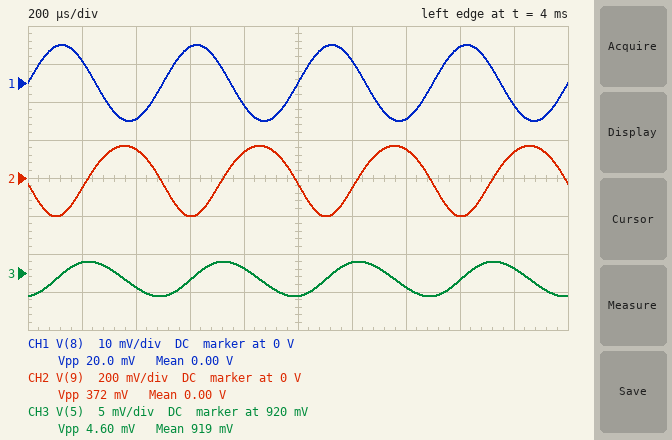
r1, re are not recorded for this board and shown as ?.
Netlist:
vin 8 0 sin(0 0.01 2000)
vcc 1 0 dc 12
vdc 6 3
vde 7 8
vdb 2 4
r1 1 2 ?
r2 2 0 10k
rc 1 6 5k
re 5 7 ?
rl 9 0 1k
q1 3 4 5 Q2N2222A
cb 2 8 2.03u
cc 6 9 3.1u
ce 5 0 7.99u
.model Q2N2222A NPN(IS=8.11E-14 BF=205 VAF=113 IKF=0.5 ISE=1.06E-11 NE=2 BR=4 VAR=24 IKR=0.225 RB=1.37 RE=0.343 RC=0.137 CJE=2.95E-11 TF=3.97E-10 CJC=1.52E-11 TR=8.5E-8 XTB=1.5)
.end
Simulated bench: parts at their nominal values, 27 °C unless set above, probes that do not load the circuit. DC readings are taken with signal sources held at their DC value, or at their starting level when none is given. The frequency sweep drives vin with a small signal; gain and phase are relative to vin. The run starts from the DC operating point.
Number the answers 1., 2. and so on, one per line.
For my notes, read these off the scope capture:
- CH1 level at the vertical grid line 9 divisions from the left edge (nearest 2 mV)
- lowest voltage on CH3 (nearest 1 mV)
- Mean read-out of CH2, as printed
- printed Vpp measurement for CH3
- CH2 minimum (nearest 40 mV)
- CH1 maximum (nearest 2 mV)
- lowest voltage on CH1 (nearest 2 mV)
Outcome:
1. -6 mV
2. 917 mV
3. 0.00 V
4. 4.60 mV
5. -200 mV
6. 10 mV
7. -10 mV
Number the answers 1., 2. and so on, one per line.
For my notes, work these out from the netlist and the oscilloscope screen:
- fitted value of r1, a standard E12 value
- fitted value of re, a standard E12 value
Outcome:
1. 68 kΩ
2. 1.5 kΩ
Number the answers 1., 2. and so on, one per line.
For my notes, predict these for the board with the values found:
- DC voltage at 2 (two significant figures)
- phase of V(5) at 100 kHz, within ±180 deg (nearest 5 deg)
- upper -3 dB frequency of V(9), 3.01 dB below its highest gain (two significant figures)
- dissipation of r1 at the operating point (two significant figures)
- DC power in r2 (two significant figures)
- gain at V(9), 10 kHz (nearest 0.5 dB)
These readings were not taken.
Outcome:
1. 1.5 V
2. -90 deg
3. 27 MHz
4. 1.6 mW
5. 230 µW
6. 25.5 dB
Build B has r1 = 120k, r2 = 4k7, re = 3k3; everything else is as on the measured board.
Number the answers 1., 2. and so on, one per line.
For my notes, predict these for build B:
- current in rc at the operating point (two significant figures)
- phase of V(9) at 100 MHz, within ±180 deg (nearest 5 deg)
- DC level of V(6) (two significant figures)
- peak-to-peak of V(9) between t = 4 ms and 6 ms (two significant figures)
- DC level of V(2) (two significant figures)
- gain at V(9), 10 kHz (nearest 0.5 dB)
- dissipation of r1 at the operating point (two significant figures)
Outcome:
1. 2.5 µA
2. 15 deg
3. 12 V
4. 1.6 mV
5. 450 mV
6. -22.0 dB
7. 1.1 mW
